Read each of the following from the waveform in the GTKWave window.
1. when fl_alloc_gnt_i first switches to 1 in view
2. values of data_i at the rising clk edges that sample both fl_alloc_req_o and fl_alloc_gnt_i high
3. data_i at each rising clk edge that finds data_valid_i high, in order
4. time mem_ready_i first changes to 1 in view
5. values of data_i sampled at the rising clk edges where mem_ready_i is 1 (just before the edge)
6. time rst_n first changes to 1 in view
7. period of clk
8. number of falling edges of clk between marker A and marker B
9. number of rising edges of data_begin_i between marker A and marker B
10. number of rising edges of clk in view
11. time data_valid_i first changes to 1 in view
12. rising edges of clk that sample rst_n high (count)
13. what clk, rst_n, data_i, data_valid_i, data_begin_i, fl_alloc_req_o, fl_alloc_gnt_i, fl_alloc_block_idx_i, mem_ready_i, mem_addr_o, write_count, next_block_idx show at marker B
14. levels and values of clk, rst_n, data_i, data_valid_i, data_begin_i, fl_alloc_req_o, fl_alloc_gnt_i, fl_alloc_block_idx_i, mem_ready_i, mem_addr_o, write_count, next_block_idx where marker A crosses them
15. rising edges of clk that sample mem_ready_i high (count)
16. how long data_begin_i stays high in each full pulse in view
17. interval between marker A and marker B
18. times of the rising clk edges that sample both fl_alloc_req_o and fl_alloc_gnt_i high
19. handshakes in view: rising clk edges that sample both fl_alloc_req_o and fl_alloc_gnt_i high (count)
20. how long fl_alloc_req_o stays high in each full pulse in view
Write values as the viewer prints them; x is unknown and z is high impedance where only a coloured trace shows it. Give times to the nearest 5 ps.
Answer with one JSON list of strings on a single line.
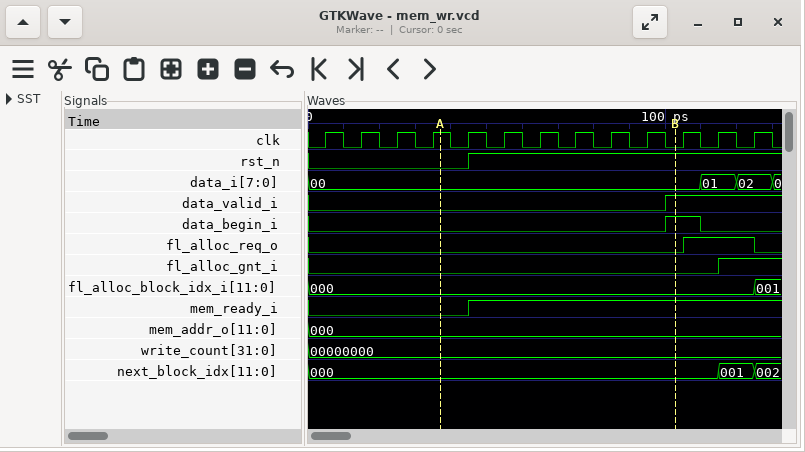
["115 ps", "02", "00, 01, 02", "45 ps", "00, 00, 00, 00, 00, 00, 01, 02", "45 ps", "10 ps", "7", "1", "13", "100 ps", "8", "clk=0, rst_n=1, data_i=00, data_valid_i=1, data_begin_i=1, fl_alloc_req_o=0, fl_alloc_gnt_i=0, fl_alloc_block_idx_i=000, mem_ready_i=1, mem_addr_o=000, write_count=00000000, next_block_idx=000", "clk=1, rst_n=0, data_i=00, data_valid_i=0, data_begin_i=0, fl_alloc_req_o=0, fl_alloc_gnt_i=0, fl_alloc_block_idx_i=000, mem_ready_i=0, mem_addr_o=000, write_count=00000000, next_block_idx=000", "8", "10 ps", "65 ps", "125 ps", "1", "20 ps"]
